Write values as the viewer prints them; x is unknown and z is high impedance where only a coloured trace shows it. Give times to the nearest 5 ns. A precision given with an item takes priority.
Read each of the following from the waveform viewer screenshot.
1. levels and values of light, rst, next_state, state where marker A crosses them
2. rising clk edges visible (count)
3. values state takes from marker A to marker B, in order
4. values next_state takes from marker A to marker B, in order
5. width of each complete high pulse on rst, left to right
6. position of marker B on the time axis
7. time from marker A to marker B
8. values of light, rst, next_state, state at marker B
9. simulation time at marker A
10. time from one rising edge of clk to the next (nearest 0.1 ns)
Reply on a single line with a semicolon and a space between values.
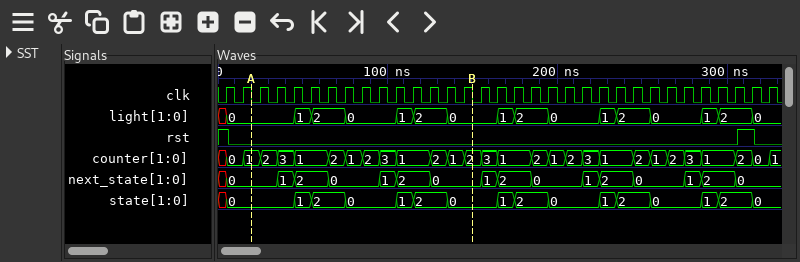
light=0, rst=0, next_state=0, state=0; 33; 0, 1, 2, 0, 1, 2, 0; 0, 1, 2, 0, 1, 2, 0; 10 ns; 150 ns; 130 ns; light=0, rst=0, next_state=0, state=0; 20 ns; 10 ns
